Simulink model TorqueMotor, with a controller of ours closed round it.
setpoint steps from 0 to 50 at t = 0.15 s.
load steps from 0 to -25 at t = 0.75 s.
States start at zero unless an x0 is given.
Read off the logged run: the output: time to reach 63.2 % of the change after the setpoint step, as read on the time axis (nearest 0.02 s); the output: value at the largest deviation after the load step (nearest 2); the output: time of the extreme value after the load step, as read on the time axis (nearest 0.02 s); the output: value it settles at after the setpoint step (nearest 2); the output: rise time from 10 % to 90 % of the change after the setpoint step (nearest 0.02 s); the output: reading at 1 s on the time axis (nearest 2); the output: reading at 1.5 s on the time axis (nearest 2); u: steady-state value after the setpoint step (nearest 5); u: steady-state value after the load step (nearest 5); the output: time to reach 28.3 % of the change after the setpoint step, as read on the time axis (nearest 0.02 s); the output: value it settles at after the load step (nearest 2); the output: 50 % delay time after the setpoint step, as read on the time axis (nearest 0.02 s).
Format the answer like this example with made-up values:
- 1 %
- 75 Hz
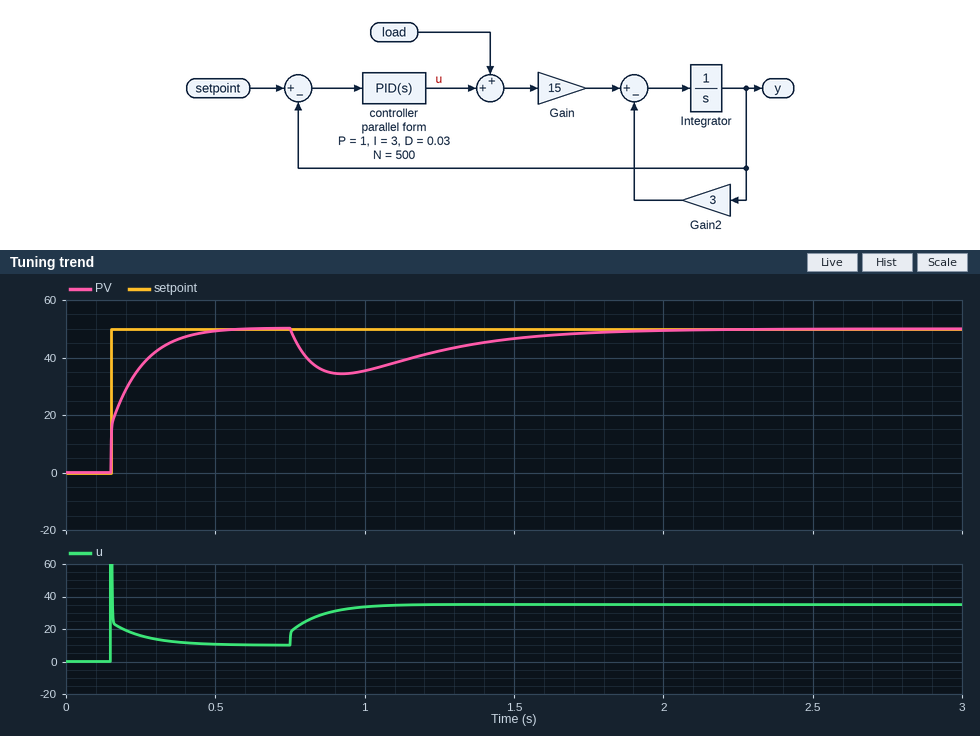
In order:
- 0.22 s
- 34
- 0.92 s
- 50
- 0.20 s
- 36
- 46
- 10
- 35
- 0.16 s
- 50
- 0.18 s
